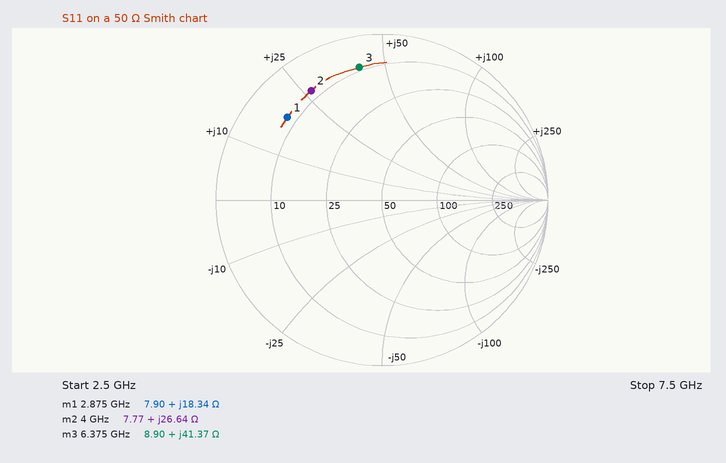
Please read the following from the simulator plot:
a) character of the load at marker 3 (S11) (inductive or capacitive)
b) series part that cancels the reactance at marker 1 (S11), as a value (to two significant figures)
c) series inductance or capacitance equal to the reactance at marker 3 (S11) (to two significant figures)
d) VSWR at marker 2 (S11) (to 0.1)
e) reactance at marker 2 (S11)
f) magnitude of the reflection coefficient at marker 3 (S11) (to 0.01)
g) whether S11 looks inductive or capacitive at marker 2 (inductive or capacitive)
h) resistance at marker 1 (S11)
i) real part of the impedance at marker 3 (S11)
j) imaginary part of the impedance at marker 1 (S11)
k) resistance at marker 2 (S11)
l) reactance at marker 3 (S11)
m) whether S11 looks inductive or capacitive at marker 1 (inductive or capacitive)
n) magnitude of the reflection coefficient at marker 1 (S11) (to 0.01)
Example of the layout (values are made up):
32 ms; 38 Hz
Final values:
inductive; 3.0 pF; 1.0 nH; 8.3; +26.64 Ω; 0.81; inductive; 7.90 Ω; 8.90 Ω; +18.34 Ω; 7.77 Ω; +41.37 Ω; inductive; 0.76
